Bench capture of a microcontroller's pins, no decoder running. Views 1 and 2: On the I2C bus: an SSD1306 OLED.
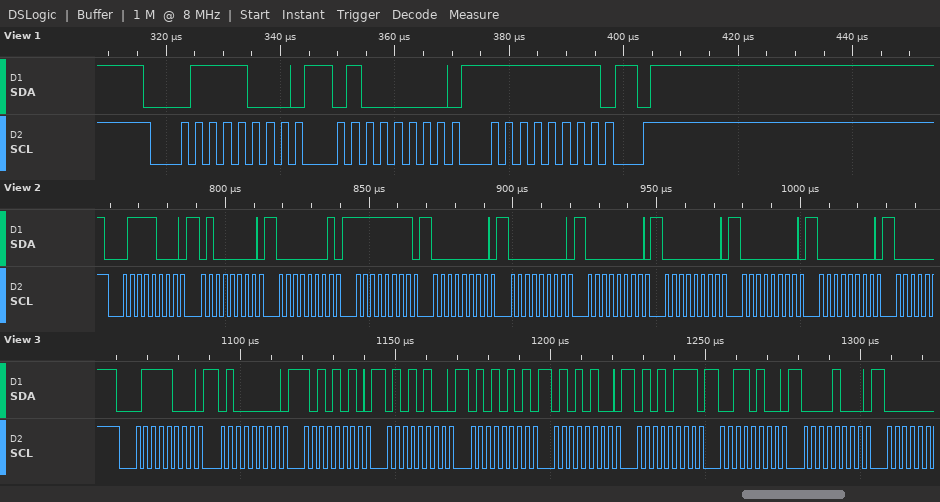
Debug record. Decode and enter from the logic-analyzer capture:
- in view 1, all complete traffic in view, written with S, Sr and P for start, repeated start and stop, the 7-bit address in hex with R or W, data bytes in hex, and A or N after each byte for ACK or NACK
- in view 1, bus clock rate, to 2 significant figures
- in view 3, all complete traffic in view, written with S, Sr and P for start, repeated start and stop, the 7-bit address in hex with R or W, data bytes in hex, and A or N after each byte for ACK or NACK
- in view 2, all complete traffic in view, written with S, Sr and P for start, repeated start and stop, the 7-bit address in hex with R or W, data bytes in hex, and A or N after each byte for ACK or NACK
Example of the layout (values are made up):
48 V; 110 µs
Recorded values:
S 3CW A 40 A FF A P; 400 kHz; S 3CW A 40 A AA A 54 A 55 A 54 A 57 A 34 A 08 A; S 3CW A 40 A 01 A FF A 00 A 00 A 00 A 00 A 00 A 00 A
